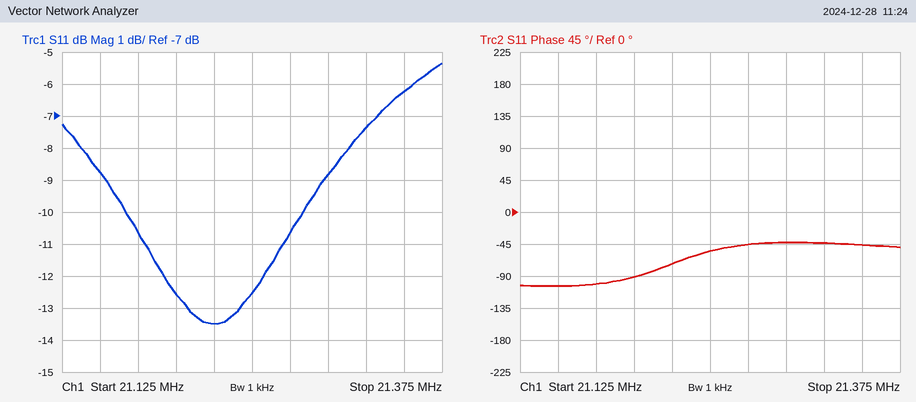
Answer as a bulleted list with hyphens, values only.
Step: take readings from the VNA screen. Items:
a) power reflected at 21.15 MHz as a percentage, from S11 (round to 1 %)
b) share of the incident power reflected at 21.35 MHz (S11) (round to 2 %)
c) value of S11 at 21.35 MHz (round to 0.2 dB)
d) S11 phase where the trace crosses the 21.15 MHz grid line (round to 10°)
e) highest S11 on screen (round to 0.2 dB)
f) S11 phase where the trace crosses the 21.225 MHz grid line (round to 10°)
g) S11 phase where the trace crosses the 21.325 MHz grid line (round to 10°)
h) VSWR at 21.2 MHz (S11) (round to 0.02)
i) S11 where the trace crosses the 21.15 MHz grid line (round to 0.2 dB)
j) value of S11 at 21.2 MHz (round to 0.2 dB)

- 13 %
- 24 %
- -6.2 dB
- -100°
- -5.4 dB
- -70°
- -40°
- 1.62
- -8.8 dB
- -12.6 dB
